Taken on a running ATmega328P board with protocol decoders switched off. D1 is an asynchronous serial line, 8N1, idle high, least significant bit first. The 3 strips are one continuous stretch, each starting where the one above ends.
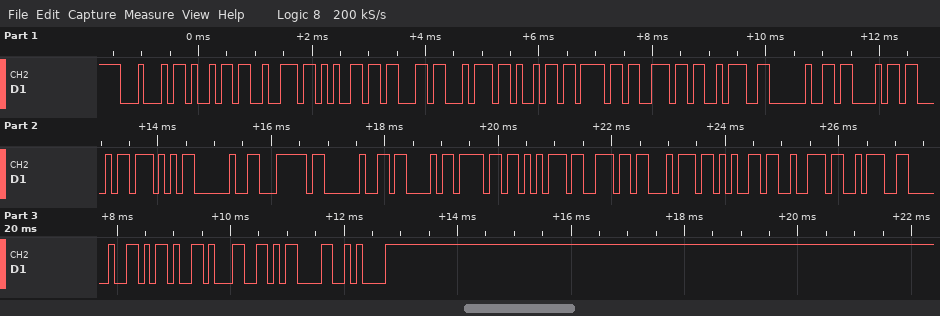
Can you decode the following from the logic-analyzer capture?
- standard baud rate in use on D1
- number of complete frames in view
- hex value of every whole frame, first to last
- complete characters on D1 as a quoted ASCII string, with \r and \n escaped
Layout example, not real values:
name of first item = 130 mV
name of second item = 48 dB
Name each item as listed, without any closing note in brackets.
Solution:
standard baud rate in use on D1 = 9600 baud
number of complete frames in view = 30
hex value of every whole frame, first to last = 44 69 72 65 63 74 69 6F 6E 3A 20 43 43 57 20 7C 20 43 6F 75 6E 74 65 72 3A 20 2D 31 0D 0A
complete characters on D1 as a quoted ASCII string, with \r and \n escaped = "Direction: CCW | Counter: -1\r\n"
